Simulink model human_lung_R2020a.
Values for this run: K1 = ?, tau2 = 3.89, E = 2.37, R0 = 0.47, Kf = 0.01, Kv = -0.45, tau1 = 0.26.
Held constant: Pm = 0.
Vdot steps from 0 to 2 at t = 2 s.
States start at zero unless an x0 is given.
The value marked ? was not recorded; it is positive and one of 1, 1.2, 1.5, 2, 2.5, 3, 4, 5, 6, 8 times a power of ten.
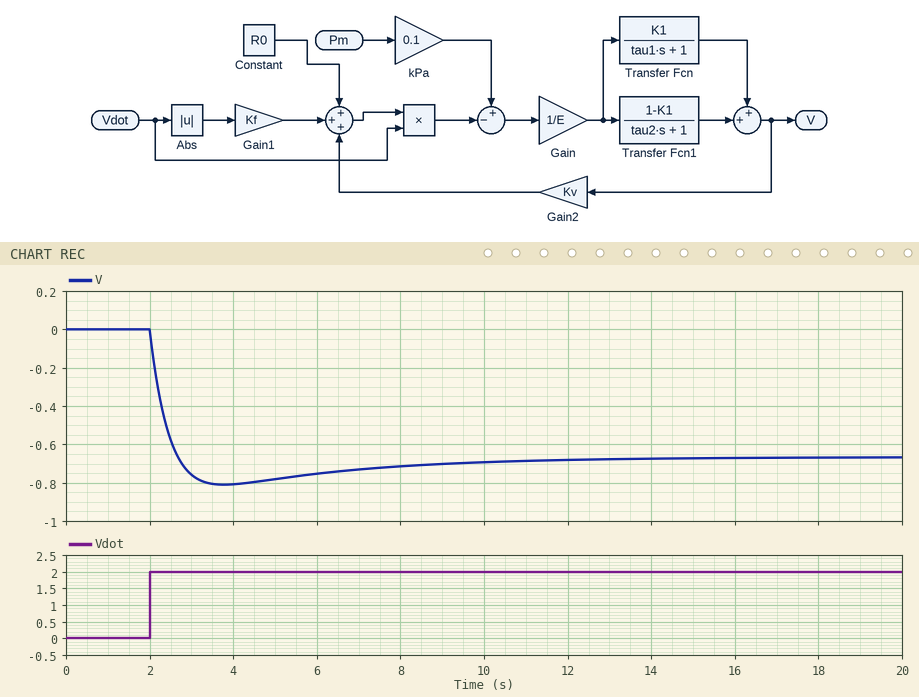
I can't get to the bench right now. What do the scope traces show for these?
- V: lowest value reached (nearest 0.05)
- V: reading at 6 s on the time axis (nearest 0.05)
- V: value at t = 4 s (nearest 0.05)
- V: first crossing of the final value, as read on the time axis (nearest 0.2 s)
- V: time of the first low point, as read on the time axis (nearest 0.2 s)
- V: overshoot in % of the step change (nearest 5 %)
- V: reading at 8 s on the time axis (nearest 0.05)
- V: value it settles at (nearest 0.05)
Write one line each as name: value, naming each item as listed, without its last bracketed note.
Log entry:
V: lowest value reached: -0.80
V: reading at 6 s on the time axis: -0.75
V: value at t = 4 s: -0.80
V: first crossing of the final value, as read on the time axis: 2.6 s
V: time of the first low point, as read on the time axis: 3.8 s
V: overshoot in % of the step change: 20 %
V: reading at 8 s on the time axis: -0.70
V: value it settles at: -0.65
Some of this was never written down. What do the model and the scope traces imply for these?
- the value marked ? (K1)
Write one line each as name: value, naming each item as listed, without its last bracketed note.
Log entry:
the value marked ?: 1.2
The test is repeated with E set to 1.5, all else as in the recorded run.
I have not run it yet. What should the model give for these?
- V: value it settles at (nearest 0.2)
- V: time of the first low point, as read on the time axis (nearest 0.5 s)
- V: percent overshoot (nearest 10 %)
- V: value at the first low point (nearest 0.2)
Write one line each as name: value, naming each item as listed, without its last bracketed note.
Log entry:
V: value it settles at: -1.6
V: time of the first low point, as read on the time axis: 4.5 s
V: percent overshoot: 30 %
V: value at the first low point: -2.2
